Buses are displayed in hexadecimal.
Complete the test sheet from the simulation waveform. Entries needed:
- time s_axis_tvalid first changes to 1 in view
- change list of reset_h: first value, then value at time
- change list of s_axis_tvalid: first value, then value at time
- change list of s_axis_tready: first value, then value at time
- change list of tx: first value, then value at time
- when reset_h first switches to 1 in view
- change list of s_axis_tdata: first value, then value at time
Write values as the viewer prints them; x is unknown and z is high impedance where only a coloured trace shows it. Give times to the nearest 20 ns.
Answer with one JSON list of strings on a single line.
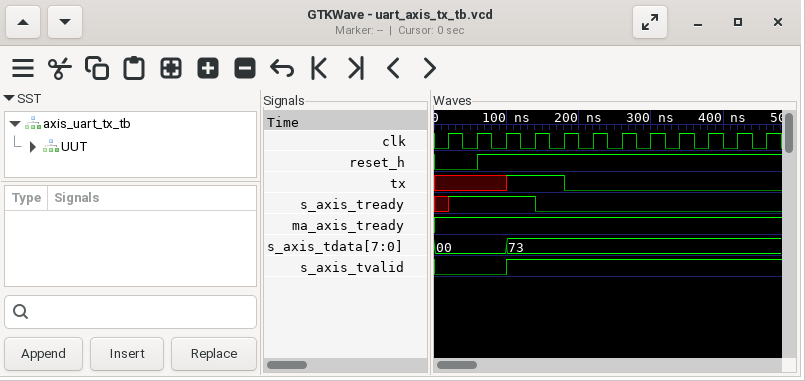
["100 ns", "0, 1 at 60 ns", "0, 1 at 100 ns", "x, 1 at 20 ns, 0 at 140 ns", "x, 1 at 100 ns, 0 at 180 ns", "60 ns", "00, 73 at 100 ns"]
